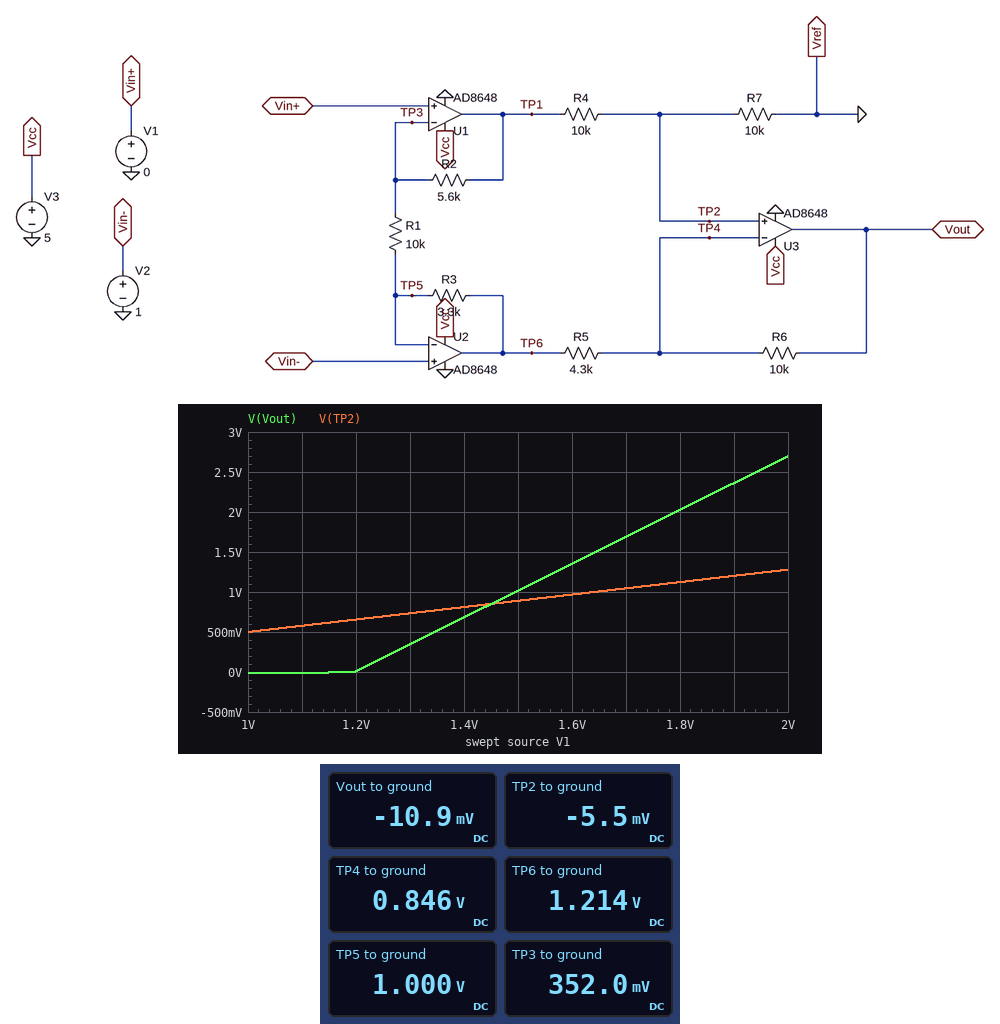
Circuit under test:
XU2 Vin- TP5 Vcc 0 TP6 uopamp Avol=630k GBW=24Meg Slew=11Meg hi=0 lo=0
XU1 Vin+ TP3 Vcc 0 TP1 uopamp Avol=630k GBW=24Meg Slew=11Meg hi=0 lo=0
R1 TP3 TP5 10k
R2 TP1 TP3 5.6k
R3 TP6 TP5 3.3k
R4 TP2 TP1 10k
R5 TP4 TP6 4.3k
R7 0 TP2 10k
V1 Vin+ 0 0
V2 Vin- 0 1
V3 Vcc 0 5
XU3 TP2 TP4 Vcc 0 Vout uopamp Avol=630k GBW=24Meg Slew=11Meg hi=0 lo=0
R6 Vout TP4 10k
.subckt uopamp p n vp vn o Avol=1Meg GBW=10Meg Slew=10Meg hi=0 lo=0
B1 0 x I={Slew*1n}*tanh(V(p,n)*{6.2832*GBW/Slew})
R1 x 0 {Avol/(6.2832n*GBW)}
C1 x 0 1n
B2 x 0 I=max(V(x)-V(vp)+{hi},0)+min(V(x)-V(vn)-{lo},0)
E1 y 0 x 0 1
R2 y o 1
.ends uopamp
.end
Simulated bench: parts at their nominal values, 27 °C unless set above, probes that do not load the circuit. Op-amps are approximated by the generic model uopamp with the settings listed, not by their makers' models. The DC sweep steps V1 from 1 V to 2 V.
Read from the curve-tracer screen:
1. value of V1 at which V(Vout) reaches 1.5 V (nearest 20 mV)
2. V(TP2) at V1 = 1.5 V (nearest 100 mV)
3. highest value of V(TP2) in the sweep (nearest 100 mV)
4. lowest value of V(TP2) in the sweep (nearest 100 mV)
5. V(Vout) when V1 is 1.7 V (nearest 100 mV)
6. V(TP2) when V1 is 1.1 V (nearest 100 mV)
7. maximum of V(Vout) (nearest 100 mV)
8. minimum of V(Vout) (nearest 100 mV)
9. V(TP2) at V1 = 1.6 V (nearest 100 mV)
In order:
1.64 V
900 mV
1.3 V
500 mV
1.7 V
600 mV
2.7 V
0 V
1.0 V
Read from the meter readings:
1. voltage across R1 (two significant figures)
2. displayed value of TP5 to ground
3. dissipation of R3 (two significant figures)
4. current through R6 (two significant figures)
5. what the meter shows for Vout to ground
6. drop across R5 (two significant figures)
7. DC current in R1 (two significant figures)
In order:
650 mV
1.000 V
14 µW
86 µA
-10.9 mV
370 mV
65 µA
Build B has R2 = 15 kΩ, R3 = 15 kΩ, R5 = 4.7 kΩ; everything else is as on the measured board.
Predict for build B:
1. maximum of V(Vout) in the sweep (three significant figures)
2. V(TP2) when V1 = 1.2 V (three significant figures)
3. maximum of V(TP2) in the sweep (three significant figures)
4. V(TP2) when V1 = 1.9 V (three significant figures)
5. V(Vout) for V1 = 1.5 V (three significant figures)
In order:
5.00 V
750 mV
1.60 V
1.52 V
2.99 V
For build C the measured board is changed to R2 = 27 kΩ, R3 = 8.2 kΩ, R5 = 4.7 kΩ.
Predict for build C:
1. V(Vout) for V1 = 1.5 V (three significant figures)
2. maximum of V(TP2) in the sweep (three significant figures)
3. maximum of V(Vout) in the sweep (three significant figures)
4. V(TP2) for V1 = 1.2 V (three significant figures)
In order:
3.20 V
2.35 V
5.01 V
870 mV
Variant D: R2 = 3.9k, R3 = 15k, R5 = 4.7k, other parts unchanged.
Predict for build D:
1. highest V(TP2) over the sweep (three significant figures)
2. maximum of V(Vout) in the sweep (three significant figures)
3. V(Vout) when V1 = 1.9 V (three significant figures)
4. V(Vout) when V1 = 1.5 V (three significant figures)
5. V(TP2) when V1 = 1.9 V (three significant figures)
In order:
1.16 V
3.64 V
3.46 V
2.12 V
1.10 V
